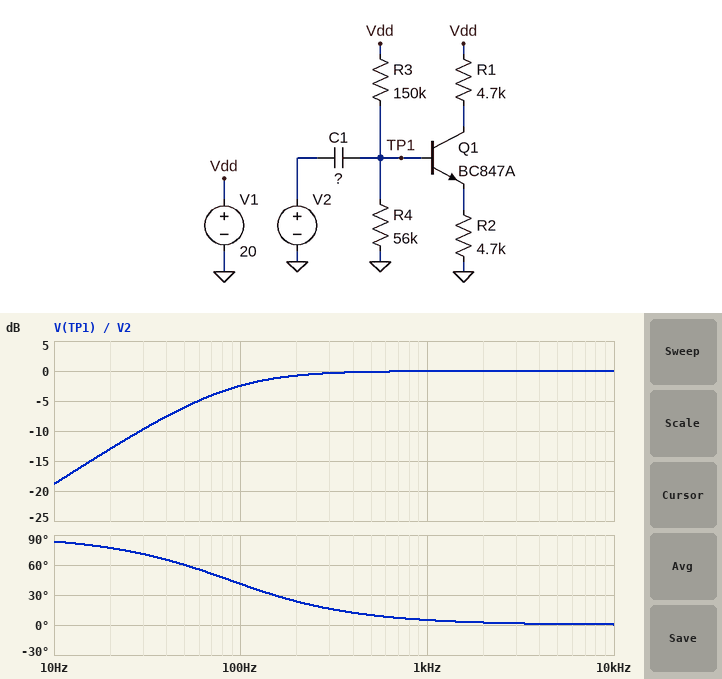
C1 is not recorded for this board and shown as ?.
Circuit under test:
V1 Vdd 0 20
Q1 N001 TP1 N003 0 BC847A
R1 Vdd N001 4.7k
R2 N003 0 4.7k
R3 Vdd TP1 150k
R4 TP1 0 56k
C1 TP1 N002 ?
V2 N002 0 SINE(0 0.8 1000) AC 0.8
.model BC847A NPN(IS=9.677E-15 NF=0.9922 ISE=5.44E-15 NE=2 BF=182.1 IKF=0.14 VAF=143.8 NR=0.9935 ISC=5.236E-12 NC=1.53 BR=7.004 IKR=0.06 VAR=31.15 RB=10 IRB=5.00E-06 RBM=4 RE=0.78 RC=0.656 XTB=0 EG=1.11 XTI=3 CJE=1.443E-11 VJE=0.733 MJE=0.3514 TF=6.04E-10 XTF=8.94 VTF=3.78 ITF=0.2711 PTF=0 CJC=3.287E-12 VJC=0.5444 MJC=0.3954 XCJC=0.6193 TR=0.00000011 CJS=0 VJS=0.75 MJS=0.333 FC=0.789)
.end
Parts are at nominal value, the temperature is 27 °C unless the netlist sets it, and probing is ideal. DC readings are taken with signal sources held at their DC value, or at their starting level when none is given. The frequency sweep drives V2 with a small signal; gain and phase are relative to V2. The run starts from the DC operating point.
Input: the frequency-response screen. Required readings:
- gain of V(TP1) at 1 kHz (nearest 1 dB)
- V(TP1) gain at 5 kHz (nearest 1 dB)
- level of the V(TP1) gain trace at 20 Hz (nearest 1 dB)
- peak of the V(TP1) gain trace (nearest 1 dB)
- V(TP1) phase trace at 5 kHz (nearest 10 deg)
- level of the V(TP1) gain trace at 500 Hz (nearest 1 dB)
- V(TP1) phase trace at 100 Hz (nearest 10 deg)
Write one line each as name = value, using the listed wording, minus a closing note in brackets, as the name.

gain of V(TP1) at 1 kHz = 0 dB
V(TP1) gain at 5 kHz = 0 dB
level of the V(TP1) gain trace at 20 Hz = -13 dB
peak of the V(TP1) gain trace = 0 dB
V(TP1) phase trace at 5 kHz = 0 deg
level of the V(TP1) gain trace at 500 Hz = 0 dB
V(TP1) phase trace at 100 Hz = 40 deg
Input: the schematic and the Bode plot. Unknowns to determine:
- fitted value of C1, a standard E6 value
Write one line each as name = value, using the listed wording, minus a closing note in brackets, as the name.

fitted value of C1, a standard E6 value = 47 nF
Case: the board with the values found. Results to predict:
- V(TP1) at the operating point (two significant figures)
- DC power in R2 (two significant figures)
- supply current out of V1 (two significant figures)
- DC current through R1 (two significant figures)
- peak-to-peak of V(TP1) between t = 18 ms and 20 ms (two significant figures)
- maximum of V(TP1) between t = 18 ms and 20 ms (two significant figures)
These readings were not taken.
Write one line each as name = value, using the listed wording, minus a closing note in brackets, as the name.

V(TP1) at the operating point = 5.2 V
DC power in R2 = 4.5 mW
supply current out of V1 = 1.1 mA
DC current through R1 = 970 µA
peak-to-peak of V(TP1) between t = 18 ms and 20 ms = 1.6 V
maximum of V(TP1) between t = 18 ms and 20 ms = 6.0 V
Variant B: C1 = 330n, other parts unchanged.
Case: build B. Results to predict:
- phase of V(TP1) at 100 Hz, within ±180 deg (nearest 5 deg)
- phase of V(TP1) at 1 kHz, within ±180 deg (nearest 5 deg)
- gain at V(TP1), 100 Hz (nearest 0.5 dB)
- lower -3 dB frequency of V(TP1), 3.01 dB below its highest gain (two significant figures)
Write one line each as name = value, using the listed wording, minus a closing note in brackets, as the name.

phase of V(TP1) at 100 Hz, within ±180 deg = 5 deg
phase of V(TP1) at 1 kHz, within ±180 deg = 0 deg
gain at V(TP1), 100 Hz = 0 dB
lower -3 dB frequency of V(TP1), 3.01 dB below its highest gain = 12 Hz
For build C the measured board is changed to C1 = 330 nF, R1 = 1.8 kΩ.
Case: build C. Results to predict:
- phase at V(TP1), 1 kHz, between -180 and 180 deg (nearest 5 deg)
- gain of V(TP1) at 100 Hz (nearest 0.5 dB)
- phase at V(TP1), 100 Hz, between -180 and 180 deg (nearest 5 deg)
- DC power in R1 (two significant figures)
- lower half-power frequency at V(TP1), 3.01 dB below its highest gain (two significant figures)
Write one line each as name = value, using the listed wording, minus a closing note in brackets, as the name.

phase at V(TP1), 1 kHz, between -180 and 180 deg = 0 deg
gain of V(TP1) at 100 Hz = 0 dB
phase at V(TP1), 100 Hz, between -180 and 180 deg = 5 deg
DC power in R1 = 1.7 mW
lower half-power frequency at V(TP1), 3.01 dB below its highest gain = 12 Hz
